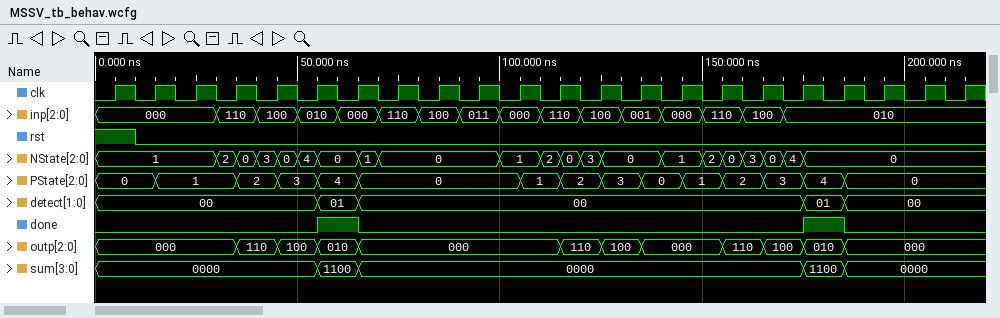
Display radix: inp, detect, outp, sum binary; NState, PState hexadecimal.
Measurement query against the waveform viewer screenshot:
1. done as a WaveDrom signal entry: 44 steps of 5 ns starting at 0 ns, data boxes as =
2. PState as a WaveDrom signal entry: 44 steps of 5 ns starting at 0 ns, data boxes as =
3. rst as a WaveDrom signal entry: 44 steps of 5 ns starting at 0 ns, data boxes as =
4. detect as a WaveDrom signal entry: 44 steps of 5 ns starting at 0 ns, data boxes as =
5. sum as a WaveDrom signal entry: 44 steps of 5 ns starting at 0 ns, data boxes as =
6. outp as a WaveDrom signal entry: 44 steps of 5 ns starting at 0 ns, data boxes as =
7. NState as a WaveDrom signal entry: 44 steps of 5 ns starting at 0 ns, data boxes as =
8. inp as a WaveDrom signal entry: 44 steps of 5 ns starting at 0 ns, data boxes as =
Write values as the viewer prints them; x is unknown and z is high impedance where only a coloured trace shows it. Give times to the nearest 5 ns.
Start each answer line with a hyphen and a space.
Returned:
- {name: 'done', wave: '0..........1.0.....................1.0......'}
- {name: 'PState', wave: '=..=...=.=.=.=.......=.=.=.=.=.=.=.=.=......', data: '0 1 2 3 4 0 1 2 3 0 1 2 3 4 0'}
- {name: 'rst', wave: '1.0.........................................'}
- {name: 'detect', wave: '=..........=.=.....................=.=......', data: '00 01 00 01 00'}
- {name: 'sum', wave: '=..........=.=.....................=.=......', data: '0000 1100 0000 1100 0000'}
- {name: 'outp', wave: '=......=.=.=.=.........=.=.=...=.=.=.=......', data: '000 110 100 010 000 110 100 000 110 100 010 000'}
- {name: 'NState', wave: '=.....======.==.....=.====..=.======........', data: '1 2 0 3 0 4 0 1 0 1 2 0 3 0 1 2 0 3 0 4 0'}
- {name: 'inp', wave: '=.....=.=.=.=.=.=.=.=.=.=.=.=.=.=.=.........', data: '000 110 100 010 000 110 100 011 000 110 100 001 000 110 100 010'}
